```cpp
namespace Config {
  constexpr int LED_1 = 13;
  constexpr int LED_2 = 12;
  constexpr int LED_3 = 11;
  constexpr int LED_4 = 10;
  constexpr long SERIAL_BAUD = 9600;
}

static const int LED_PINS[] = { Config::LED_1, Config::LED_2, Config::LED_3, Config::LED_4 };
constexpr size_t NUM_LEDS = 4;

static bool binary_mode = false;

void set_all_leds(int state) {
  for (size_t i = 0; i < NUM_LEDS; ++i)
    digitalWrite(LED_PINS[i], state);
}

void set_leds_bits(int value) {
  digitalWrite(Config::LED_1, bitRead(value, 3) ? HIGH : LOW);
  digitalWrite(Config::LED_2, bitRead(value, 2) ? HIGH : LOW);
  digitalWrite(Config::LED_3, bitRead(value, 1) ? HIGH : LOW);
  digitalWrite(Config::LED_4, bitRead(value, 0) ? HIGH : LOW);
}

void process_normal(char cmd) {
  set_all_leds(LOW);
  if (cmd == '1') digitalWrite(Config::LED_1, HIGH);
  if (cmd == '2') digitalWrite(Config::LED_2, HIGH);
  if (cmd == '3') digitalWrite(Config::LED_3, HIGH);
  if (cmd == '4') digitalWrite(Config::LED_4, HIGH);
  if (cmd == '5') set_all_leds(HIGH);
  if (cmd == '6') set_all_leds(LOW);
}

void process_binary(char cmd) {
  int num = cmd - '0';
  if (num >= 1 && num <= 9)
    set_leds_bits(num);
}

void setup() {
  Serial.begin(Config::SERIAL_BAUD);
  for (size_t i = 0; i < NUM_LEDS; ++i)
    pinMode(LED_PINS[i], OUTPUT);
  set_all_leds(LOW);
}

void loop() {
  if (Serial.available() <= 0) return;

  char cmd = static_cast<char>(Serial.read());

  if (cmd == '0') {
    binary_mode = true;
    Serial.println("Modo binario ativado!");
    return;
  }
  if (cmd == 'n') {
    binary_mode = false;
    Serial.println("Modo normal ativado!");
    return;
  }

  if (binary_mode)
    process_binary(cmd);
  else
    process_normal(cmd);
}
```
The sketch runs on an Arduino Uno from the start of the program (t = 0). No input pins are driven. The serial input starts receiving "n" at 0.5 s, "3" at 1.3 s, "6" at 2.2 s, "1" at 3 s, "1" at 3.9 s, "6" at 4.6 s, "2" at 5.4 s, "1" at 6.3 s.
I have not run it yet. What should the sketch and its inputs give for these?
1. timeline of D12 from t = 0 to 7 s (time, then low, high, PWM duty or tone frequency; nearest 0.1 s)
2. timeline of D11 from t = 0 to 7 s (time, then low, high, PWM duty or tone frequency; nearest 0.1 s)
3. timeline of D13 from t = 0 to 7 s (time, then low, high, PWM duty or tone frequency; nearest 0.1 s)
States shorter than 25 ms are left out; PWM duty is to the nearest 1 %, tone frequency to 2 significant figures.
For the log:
0 s low; 5.4 s high; 6.3 s low
0 s low; 1.3 s high; 2.2 s low
0 s low; 3 s high; 4.6 s low; 6.3 s high
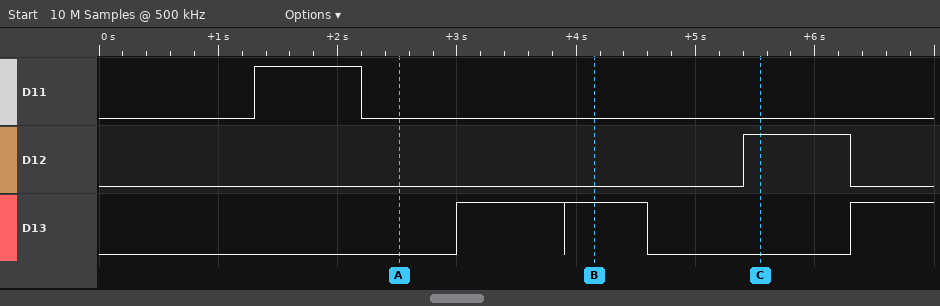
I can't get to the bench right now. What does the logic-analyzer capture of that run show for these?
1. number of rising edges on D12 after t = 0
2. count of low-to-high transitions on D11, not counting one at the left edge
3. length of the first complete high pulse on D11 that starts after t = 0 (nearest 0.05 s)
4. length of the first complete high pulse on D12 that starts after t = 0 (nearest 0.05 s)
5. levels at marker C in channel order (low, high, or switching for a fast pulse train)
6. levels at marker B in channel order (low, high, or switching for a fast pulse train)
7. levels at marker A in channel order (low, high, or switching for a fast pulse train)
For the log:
1
1
0.90 s
0.90 s
D11 low, D12 high, D13 low
D11 low, D12 low, D13 high
D11 low, D12 low, D13 low
